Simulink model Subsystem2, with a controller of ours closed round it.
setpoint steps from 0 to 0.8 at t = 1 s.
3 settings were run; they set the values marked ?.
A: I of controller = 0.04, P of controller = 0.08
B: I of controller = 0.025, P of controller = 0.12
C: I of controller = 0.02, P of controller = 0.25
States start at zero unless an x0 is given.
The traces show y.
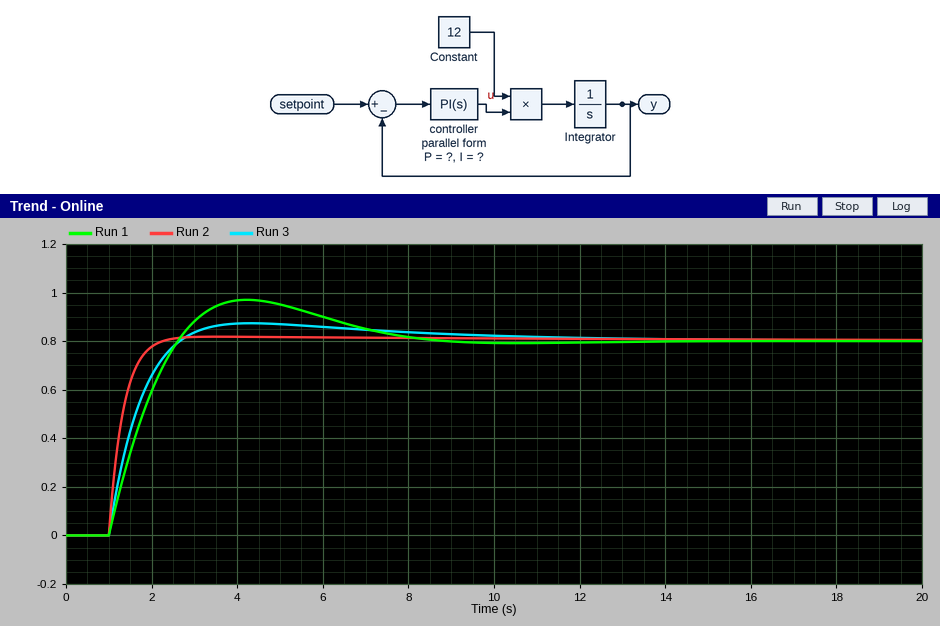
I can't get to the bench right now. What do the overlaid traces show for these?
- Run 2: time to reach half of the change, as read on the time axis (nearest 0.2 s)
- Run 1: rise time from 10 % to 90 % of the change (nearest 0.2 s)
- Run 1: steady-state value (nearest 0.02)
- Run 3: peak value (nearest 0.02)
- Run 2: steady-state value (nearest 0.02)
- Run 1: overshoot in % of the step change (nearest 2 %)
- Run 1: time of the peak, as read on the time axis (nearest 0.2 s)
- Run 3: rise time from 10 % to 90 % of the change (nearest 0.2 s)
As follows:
1.2 s
1.2 s
0.80
0.88
0.80
22 %
4.2 s
1.2 s
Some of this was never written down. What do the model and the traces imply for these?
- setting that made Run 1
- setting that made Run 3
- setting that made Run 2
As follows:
A
B
C
